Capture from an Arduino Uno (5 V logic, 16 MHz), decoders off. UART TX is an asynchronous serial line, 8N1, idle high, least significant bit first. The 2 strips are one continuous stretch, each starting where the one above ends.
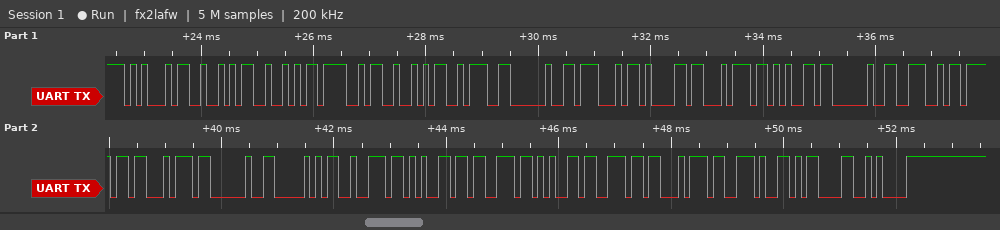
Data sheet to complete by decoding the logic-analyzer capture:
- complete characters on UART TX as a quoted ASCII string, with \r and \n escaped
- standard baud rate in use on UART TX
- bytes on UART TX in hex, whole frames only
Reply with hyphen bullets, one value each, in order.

- "ERROR: Gate Not Present.\r\n"
- 9600 baud
- 45 52 52 4F 52 3A 20 47 61 74 65 20 4E 6F 74 20 50 72 65 73 65 6E 74 2E 0D 0A
